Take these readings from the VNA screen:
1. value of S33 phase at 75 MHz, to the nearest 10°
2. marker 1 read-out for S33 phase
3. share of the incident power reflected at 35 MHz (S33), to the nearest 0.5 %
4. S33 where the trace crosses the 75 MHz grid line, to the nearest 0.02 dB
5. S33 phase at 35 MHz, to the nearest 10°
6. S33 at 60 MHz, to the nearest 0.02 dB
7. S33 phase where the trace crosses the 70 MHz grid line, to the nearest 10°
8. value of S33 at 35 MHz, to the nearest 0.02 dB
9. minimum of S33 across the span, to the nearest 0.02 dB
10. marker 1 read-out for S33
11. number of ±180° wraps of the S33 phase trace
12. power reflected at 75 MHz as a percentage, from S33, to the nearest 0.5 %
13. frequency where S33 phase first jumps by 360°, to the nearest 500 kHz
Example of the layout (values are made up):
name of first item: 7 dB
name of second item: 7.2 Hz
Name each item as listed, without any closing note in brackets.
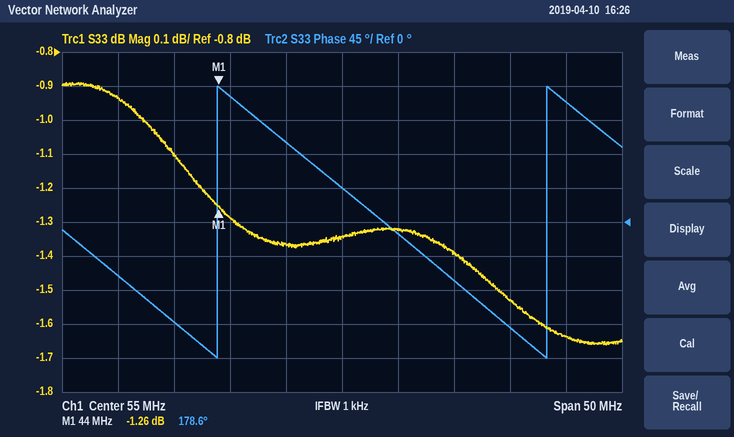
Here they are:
value of S33 phase at 75 MHz, to the nearest 10°: 160°
marker 1 read-out for S33 phase: 178.6°
share of the incident power reflected at 35 MHz (S33), to the nearest 0.5 %: 80.5 %
S33 where the trace crosses the 75 MHz grid line, to the nearest 0.02 dB: -1.64 dB
S33 phase at 35 MHz, to the nearest 10°: -70°
S33 at 60 MHz, to the nearest 0.02 dB: -1.32 dB
S33 phase where the trace crosses the 70 MHz grid line, to the nearest 10°: -140°
value of S33 at 35 MHz, to the nearest 0.02 dB: -0.94 dB
minimum of S33 across the span, to the nearest 0.02 dB: -1.66 dB
marker 1 read-out for S33: -1.26 dB
number of ±180° wraps of the S33 phase trace: 2
power reflected at 75 MHz as a percentage, from S33, to the nearest 0.5 %: 68.5 %
frequency where S33 phase first jumps by 360°, to the nearest 500 kHz: 44.0 MHz
